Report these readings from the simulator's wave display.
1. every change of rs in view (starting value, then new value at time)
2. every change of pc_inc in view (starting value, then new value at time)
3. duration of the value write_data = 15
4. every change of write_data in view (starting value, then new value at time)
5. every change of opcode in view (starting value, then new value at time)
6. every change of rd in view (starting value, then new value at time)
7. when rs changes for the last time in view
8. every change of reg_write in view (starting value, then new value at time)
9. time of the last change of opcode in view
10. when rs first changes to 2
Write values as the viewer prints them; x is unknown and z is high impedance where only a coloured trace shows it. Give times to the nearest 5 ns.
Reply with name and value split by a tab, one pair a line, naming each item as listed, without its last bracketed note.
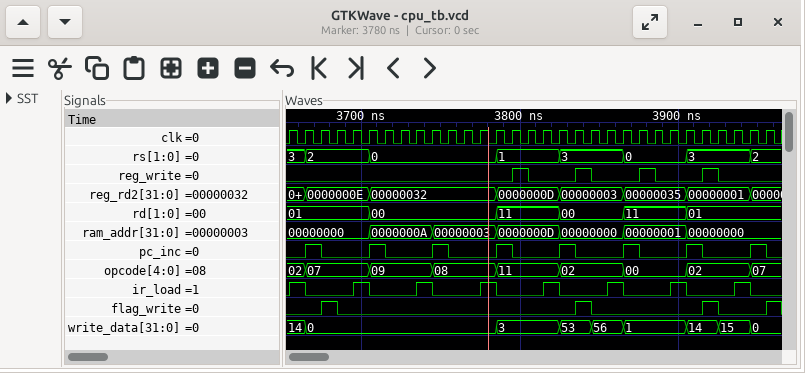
every change of rs in view	3, 2 at 3665 ns, 0 at 3705 ns, 1 at 3785 ns, 3 at 3825 ns, 0 at 3865 ns, 3 at 3905 ns, 2 at 3945 ns
every change of pc_inc in view	0, 1 at 3665 ns, 0 at 3675 ns, 1 at 3705 ns, 0 at 3715 ns, 1 at 3745 ns, 0 at 3755 ns, 1 at 3785 ns, 0 at 3795 ns, 1 at 3825 ns, 0 at 3835 ns, 1 at 3865 ns, 0 at 3875 ns, 1 at 3905 ns, 0 at 3915 ns, 1 at 3945 ns, 0 at 3955 ns
duration of the value write_data = 15	20 ns
every change of write_data in view	14, 0 at 3665 ns, 3 at 3785 ns, 53 at 3825 ns, 56 at 3845 ns, 1 at 3865 ns, 14 at 3905 ns, 15 at 3925 ns, 0 at 3945 ns
every change of opcode in view	02, 07 at 3665 ns, 09 at 3705 ns, 08 at 3745 ns, 11 at 3785 ns, 02 at 3825 ns, 00 at 3865 ns, 02 at 3905 ns, 07 at 3945 ns
every change of rd in view	01, 00 at 3705 ns, 11 at 3785 ns, 00 at 3825 ns, 11 at 3865 ns, 01 at 3905 ns
when rs changes for the last time in view	3945 ns
every change of reg_write in view	0, 1 at 3795 ns, 0 at 3805 ns, 1 at 3835 ns, 0 at 3845 ns, 1 at 3875 ns, 0 at 3885 ns, 1 at 3915 ns, 0 at 3925 ns
time of the last change of opcode in view	3945 ns
when rs first changes to 2	3665 ns
